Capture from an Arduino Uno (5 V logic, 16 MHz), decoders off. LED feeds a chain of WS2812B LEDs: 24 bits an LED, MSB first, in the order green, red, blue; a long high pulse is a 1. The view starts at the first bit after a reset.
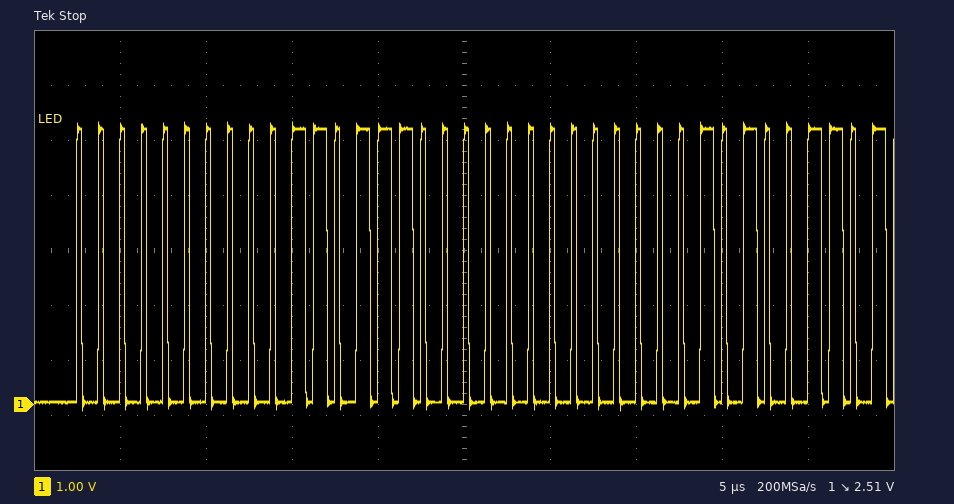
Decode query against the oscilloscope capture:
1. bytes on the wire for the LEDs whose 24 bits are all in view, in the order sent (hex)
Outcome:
00 37 00
